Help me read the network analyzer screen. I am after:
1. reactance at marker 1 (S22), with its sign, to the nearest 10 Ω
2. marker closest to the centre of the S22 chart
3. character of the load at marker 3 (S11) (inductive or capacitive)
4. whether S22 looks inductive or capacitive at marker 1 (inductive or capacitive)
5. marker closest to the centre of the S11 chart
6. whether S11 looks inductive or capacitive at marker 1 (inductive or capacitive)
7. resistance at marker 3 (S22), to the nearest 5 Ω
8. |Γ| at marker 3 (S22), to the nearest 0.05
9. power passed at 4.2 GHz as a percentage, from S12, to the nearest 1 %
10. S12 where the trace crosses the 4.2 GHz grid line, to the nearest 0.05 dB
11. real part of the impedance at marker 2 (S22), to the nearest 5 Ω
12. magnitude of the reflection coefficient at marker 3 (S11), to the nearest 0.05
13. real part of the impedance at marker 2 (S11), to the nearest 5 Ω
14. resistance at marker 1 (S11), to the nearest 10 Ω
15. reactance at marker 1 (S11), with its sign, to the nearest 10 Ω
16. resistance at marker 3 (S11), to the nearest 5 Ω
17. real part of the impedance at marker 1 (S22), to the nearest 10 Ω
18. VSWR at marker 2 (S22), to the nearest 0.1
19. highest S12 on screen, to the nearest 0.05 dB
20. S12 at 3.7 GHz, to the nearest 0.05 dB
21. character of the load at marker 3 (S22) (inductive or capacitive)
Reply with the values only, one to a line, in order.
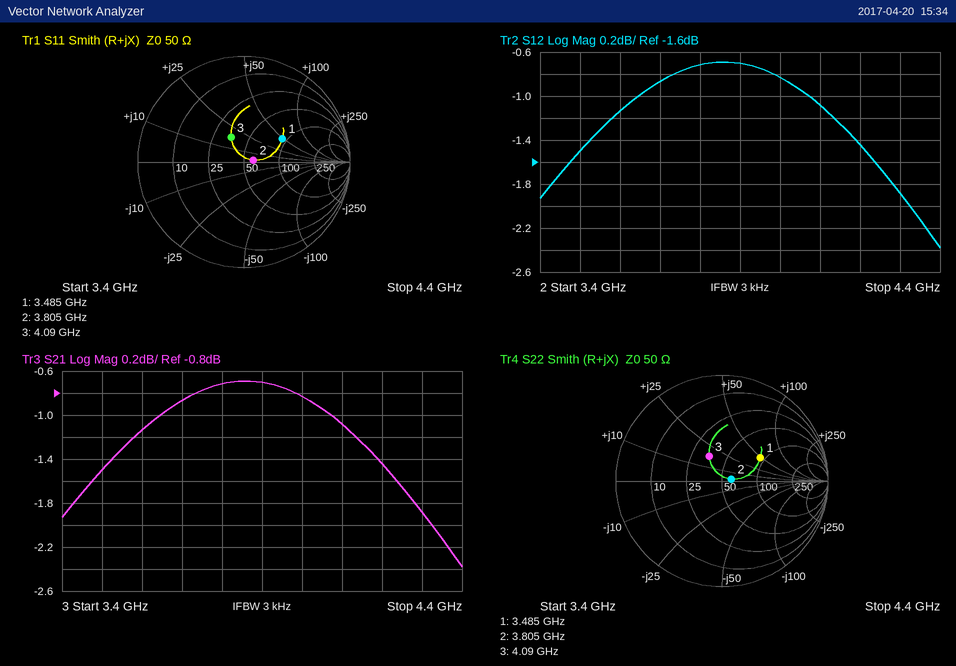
+50 Ω
marker 2
inductive
inductive
marker 2
inductive
35 Ω
0.25
72 %
-1.45 dB
60 Ω
0.25
60 Ω
90 Ω
+50 Ω
35 Ω
90 Ω
1.2
-0.70 dB
-0.85 dB
inductive
